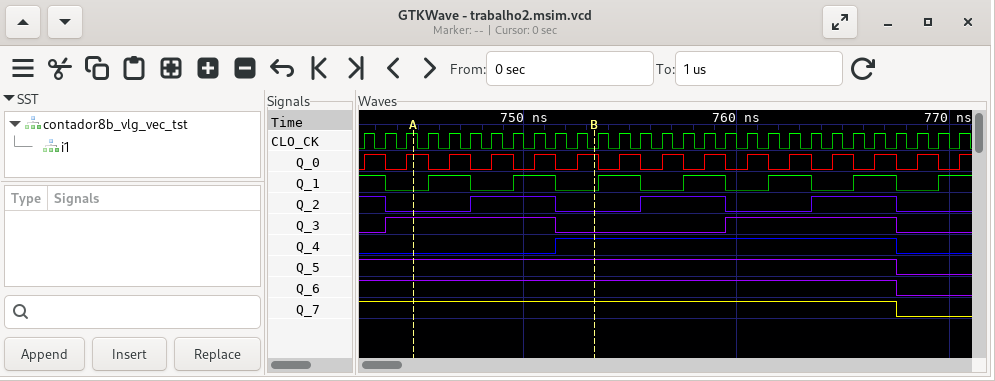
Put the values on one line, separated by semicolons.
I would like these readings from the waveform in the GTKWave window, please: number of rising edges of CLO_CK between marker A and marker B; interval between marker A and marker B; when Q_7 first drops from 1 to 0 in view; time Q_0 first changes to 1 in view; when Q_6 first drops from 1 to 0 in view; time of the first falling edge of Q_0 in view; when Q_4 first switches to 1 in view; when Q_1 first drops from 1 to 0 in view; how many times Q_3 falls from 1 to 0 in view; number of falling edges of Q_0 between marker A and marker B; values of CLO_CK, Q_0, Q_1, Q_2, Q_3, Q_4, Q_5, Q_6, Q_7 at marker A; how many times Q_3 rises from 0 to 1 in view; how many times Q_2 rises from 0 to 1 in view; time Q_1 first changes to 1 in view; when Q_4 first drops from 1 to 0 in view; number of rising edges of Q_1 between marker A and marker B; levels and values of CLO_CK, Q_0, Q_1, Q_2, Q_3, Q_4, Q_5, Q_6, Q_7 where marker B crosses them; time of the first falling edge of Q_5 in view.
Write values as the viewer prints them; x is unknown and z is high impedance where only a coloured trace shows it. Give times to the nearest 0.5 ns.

8; 8.5 ns; 767.5 ns; 742.5 ns; 767.5 ns; 743.5 ns; 751.5 ns; 743.5 ns; 2; 4; CLO_CK=1, Q_0=1, Q_1=0, Q_2=0, Q_3=1, Q_4=0, Q_5=1, Q_6=1, Q_7=1; 2; 3; 745.5 ns; 767.5 ns; 2; CLO_CK=0, Q_0=1, Q_1=0, Q_2=0, Q_3=0, Q_4=1, Q_5=1, Q_6=1, Q_7=1; 767.5 ns
